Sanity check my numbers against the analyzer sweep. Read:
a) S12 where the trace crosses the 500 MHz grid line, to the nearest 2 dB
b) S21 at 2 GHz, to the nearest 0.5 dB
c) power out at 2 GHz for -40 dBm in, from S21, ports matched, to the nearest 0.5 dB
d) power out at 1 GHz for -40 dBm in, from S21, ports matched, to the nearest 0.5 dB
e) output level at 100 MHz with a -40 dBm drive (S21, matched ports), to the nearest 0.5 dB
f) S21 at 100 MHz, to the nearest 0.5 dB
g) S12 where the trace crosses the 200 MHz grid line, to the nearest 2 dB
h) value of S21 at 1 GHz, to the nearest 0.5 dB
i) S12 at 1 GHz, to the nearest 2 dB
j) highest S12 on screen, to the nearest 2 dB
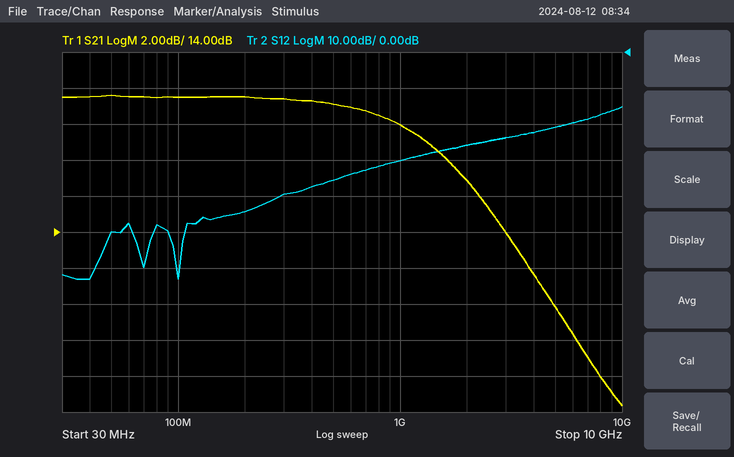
-36 dB
17.0 dB
-23.0 dBm
-20.0 dBm
-18.5 dBm
21.5 dB
-44 dB
20.0 dB
-30 dB
-16 dB
